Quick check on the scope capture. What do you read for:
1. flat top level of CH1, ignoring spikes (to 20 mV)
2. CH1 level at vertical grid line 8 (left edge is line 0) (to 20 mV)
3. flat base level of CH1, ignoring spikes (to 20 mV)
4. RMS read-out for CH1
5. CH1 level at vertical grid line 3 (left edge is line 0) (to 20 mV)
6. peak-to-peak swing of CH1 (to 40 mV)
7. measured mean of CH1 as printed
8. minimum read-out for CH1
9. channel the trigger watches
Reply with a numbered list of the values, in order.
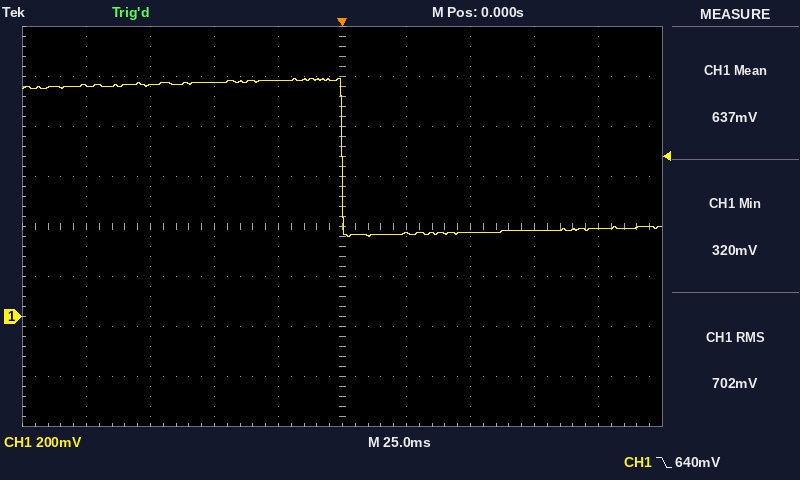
1. 940 mV
2. 340 mV
3. 340 mV
4. 702 mV
5. 940 mV
6. 640 mV
7. 637 mV
8. 320 mV
9. CH1
